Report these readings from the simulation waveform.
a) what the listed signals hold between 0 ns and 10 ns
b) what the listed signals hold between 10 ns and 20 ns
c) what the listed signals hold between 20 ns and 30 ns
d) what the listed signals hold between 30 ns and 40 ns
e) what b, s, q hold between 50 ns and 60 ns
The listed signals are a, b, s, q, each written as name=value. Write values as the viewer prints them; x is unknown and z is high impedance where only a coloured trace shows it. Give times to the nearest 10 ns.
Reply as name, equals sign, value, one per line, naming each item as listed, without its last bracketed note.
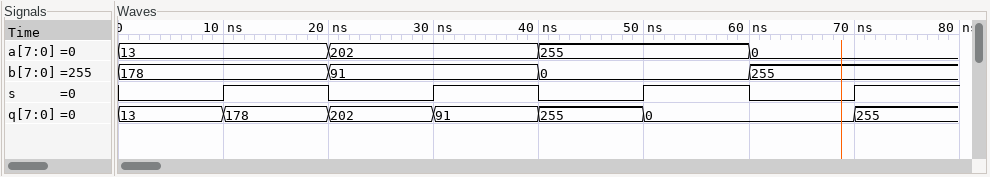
what the listed signals hold between 0 ns and 10 ns = a=13, b=178, s=0, q=13
what the listed signals hold between 10 ns and 20 ns = a=13, b=178, s=1, q=178
what the listed signals hold between 20 ns and 30 ns = a=202, b=91, s=0, q=202
what the listed signals hold between 30 ns and 40 ns = a=202, b=91, s=1, q=91
what b, s, q hold between 50 ns and 60 ns = b=0, s=1, q=0
